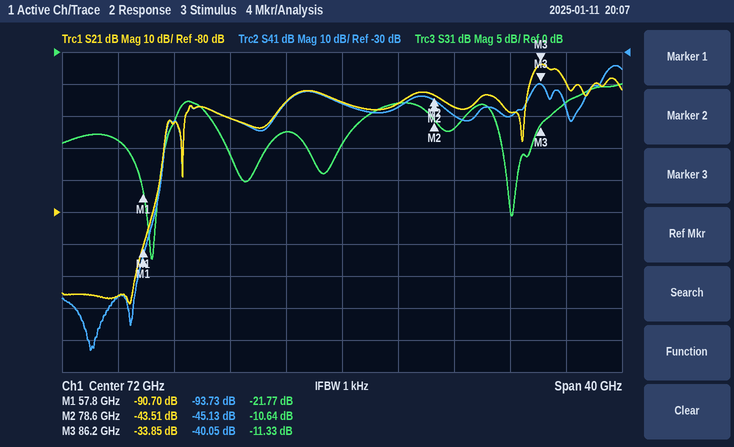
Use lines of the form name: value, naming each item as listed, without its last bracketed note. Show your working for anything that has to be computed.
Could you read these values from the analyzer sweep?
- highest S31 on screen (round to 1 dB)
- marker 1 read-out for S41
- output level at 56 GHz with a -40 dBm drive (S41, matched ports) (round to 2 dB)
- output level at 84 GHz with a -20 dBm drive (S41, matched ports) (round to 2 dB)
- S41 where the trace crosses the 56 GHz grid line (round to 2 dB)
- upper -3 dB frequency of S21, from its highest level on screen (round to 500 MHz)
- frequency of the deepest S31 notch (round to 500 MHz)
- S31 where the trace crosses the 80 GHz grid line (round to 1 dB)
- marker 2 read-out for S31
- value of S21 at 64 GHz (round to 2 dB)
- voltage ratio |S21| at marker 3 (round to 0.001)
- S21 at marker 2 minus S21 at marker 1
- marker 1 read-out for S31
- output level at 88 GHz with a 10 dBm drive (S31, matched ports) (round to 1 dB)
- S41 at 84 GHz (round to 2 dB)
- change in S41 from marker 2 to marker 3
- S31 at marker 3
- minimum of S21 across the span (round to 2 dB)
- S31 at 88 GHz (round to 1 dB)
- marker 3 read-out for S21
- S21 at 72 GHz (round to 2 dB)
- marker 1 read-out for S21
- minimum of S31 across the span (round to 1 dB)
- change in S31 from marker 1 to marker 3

highest S31 on screen: -5 dB
marker 1 read-out for S41: -93.73 dB
output level at 56 GHz with a -40 dBm drive (S41, matched ports): -40 dBm + (-106 dB) = -146 dBm
output level at 84 GHz with a -20 dBm drive (S41, matched ports): -20 dBm + (-50 dB) = -70 dBm
S41 where the trace crosses the 56 GHz grid line: -106 dB
upper -3 dB frequency of S21, from its highest level on screen: 87.5 GHz
frequency of the deepest S31 notch: 58.5 GHz
S31 where the trace crosses the 80 GHz grid line: -12 dB
marker 2 read-out for S31: -10.64 dB
value of S21 at 64 GHz: -50 dB
voltage ratio |S21| at marker 3: 10^(-33.85/20) ≈ 0.020
S21 at marker 2 minus S21 at marker 1: -43.51 − (-90.7) = 47.19 dB
marker 1 read-out for S31: -21.77 dB
output level at 88 GHz with a 10 dBm drive (S31, matched ports): 10 dBm + (-8 dB) = 2 dBm
S41 at 84 GHz: -50 dB
change in S41 from marker 2 to marker 3: -40.05 − (-45.13) = 5.08 dB
S31 at marker 3: -11.33 dB
minimum of S21 across the span: -108 dB
S31 at 88 GHz: -8 dB
marker 3 read-out for S21: -33.85 dB
S21 at 72 GHz: -46 dB
marker 1 read-out for S21: -90.70 dB
minimum of S31 across the span: -32 dB
change in S31 from marker 1 to marker 3: -11.33 − (-21.77) = 10.44 dB
